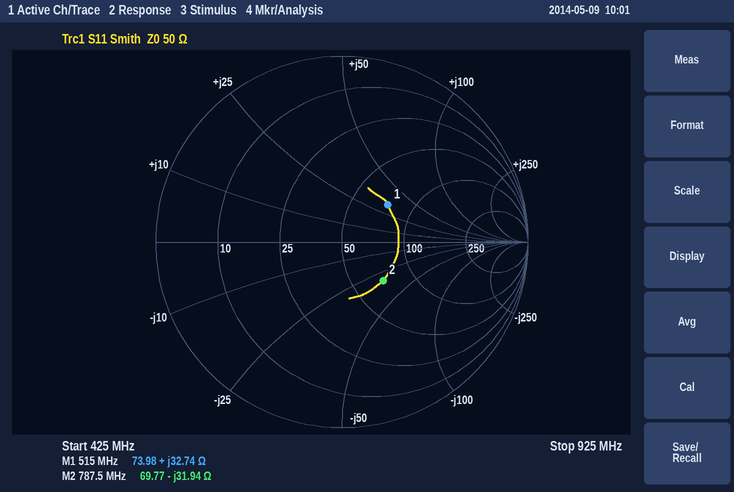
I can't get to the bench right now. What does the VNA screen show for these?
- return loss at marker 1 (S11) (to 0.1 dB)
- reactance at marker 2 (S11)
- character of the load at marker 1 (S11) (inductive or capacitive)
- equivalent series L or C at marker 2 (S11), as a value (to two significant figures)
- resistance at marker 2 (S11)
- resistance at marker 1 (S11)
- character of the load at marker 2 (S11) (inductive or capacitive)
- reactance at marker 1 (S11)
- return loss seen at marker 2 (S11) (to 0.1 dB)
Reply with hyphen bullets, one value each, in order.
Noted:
- 10.0 dB
- -31.94 Ω
- inductive
- 6.3 pF
- 69.77 Ω
- 73.98 Ω
- capacitive
- +32.74 Ω
- 10.4 dB
